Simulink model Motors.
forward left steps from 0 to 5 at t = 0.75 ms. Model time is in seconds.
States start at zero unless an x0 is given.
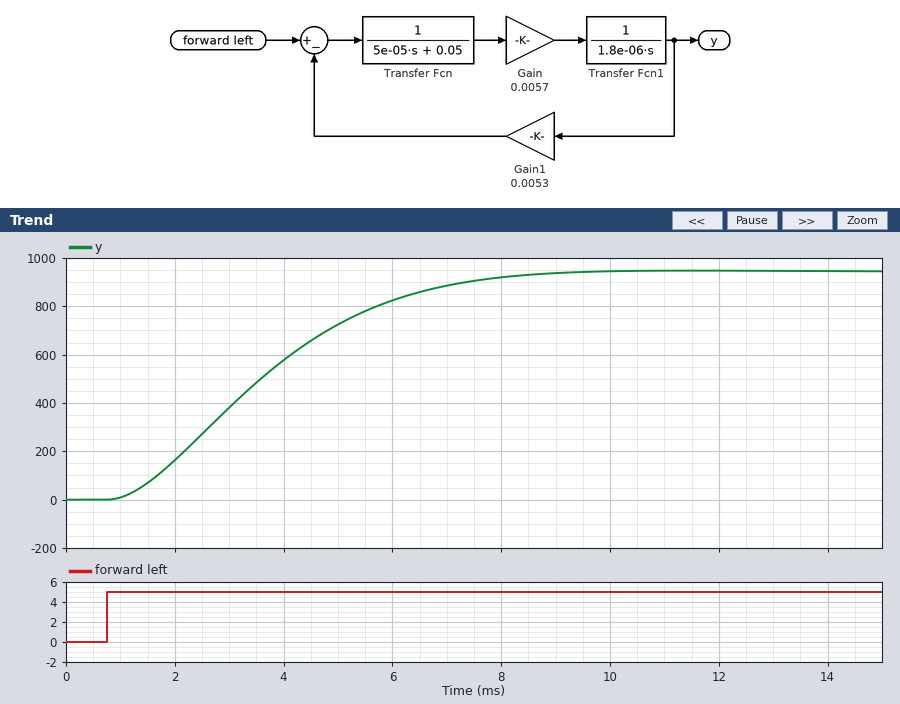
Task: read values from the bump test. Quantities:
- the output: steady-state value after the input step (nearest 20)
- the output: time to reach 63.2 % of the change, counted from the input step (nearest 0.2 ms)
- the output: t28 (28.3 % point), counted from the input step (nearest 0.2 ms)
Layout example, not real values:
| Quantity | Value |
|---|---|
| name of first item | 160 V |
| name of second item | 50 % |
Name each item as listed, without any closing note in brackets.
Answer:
| Quantity | Value |
|---|---|
| the output: steady-state value after the input step | 940 |
| the output: time to reach 63.2 % of the change, counted from the input step | 3.4 ms |
| the output: t28 (28.3 % point), counted from the input step | 1.8 ms |
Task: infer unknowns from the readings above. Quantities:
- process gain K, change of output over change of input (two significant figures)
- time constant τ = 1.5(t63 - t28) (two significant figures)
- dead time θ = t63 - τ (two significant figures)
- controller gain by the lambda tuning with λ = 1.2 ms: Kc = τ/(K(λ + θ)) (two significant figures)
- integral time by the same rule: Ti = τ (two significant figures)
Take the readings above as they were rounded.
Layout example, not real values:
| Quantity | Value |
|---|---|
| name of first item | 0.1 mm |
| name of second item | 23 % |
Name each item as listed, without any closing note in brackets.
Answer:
| Quantity | Value |
|---|---|
| process gain K, change of output over change of input | 190 |
| time constant τ = 1.5(t63 - t28) | 2.4 ms |
| dead time θ = t63 - τ | 1.0 ms |
| controller gain by the lambda tuning with λ = 1.2 ms: Kc = τ/(K(λ + θ)) | 0.0057 |
| integral time by the same rule: Ti = τ | 2.4 ms |
